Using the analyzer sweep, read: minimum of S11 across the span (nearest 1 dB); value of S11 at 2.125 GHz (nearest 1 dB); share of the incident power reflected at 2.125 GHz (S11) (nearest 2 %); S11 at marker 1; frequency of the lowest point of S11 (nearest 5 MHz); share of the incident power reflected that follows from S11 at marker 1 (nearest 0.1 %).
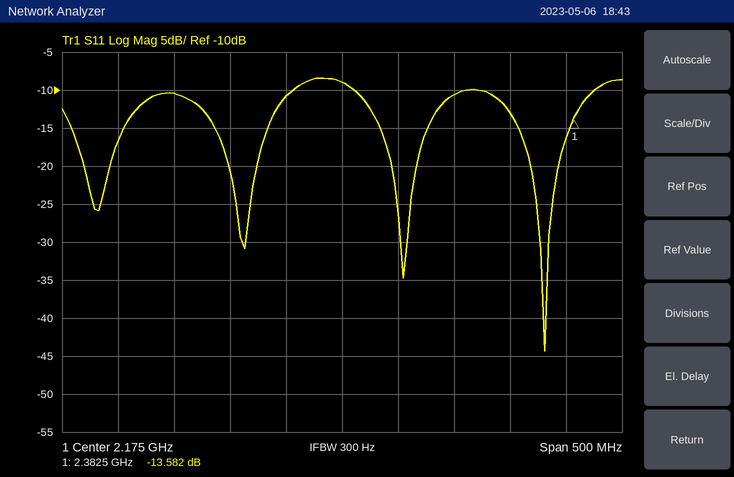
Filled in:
-44 dB
-11 dB
8 %
-13.582 dB
2.355 GHz
4.4 %
